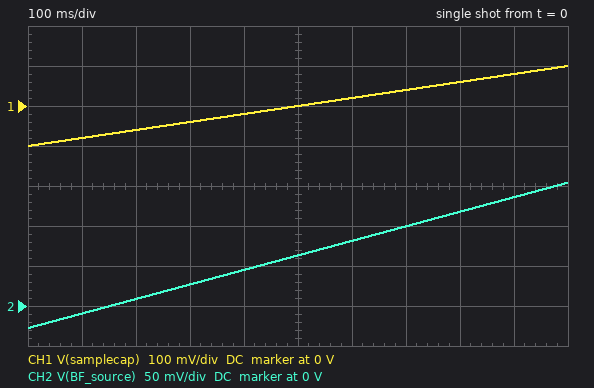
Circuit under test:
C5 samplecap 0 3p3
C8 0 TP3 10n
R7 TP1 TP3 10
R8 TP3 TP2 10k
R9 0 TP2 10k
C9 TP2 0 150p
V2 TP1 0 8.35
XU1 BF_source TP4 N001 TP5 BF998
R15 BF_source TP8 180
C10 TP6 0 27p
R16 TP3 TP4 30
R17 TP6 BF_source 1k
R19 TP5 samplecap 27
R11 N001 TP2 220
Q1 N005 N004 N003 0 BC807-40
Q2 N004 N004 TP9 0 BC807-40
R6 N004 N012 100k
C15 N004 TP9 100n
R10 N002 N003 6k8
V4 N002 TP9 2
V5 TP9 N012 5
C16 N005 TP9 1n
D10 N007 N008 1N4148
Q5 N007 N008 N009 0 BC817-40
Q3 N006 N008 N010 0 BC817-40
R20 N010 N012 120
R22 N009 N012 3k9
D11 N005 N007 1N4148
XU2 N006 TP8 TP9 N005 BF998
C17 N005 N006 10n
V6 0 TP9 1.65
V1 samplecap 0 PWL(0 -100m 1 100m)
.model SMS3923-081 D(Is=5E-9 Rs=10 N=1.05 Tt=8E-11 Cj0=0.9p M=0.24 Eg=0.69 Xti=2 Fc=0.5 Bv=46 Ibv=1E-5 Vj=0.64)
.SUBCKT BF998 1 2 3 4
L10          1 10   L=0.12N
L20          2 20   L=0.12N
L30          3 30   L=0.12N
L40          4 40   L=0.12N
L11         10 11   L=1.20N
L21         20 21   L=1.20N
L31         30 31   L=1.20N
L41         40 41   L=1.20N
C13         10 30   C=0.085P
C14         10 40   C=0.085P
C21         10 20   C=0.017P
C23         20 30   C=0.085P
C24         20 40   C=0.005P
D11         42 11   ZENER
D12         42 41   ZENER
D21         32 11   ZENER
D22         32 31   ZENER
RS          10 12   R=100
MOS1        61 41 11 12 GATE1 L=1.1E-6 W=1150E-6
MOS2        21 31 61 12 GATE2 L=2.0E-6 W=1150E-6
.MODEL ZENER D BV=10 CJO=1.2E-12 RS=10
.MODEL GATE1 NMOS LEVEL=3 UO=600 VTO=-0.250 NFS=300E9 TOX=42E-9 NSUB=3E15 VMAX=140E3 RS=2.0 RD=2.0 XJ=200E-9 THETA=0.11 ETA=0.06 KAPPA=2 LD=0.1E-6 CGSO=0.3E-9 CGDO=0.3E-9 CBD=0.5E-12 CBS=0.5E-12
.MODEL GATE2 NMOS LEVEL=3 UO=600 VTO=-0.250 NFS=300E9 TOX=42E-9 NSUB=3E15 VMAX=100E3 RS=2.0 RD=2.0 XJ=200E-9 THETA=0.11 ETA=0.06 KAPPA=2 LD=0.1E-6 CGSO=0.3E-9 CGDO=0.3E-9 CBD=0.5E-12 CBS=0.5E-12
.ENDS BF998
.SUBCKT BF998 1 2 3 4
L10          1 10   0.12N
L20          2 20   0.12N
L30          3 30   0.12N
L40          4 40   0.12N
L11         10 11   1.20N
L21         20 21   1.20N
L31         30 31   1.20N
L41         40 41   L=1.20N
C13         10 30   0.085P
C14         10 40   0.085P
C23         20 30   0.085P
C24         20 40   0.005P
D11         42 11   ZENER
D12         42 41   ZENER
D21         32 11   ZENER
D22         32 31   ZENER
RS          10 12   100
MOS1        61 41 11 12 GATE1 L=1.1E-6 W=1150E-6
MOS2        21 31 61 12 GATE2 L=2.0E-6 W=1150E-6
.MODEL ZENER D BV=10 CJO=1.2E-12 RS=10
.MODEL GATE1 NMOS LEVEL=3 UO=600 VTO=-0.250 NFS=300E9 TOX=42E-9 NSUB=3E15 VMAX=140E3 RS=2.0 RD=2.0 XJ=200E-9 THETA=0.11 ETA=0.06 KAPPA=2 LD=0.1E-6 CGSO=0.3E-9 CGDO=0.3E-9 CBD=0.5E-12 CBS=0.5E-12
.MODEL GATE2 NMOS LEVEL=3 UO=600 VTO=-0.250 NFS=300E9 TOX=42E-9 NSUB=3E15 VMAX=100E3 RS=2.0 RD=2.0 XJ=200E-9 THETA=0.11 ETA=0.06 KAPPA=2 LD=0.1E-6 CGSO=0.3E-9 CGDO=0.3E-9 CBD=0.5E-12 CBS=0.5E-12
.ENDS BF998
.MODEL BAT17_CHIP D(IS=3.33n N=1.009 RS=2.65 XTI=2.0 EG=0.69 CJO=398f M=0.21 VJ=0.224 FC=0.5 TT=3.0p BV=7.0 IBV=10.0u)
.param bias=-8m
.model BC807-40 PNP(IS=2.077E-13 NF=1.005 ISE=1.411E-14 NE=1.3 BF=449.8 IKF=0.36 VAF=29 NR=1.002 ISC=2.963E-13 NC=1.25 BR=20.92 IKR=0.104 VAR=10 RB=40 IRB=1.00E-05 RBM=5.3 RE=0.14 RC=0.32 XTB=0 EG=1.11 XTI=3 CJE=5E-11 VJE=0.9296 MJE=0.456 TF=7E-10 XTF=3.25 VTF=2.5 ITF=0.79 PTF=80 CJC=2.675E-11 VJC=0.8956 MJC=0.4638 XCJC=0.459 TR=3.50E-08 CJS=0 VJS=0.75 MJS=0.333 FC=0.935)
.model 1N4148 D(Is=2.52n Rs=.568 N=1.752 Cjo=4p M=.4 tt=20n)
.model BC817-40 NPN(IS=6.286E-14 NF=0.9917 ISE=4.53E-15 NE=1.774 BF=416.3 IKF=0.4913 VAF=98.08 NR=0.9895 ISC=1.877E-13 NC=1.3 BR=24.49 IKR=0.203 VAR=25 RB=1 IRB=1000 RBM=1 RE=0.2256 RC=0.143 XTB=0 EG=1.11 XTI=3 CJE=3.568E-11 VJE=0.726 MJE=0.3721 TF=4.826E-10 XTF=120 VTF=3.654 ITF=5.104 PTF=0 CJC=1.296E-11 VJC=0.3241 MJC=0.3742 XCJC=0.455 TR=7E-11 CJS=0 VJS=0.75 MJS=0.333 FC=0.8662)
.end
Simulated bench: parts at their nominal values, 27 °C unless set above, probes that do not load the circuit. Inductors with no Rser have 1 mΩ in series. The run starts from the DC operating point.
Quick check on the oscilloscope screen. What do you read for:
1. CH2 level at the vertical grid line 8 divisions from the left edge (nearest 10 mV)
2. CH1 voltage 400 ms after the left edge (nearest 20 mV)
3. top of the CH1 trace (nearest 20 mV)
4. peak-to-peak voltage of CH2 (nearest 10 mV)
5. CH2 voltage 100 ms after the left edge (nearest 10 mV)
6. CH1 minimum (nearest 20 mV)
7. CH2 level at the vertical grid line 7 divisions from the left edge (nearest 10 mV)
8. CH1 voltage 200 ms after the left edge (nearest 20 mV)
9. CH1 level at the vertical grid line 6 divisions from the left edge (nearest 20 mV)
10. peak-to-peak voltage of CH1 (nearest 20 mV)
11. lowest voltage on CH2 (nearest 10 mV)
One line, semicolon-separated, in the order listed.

120 mV; -20 mV; 100 mV; 180 mV; -10 mV; -100 mV; 100 mV; -60 mV; 20 mV; 200 mV; -30 mV
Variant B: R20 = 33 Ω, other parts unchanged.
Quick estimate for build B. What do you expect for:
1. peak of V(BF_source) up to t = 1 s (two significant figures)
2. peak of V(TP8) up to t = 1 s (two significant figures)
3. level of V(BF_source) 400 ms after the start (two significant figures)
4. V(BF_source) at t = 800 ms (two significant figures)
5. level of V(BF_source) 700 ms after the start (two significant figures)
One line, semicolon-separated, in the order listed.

-330 mV; -4.5 V; -440 mV; -370 mV; -390 mV
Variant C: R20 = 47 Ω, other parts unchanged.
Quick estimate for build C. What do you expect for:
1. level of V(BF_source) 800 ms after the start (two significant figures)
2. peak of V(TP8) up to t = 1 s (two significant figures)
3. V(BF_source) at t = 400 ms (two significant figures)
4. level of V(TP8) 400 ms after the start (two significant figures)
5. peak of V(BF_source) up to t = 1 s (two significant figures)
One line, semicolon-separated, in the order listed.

-210 mV; -3.3 V; -280 mV; -3.4 V; -170 mV
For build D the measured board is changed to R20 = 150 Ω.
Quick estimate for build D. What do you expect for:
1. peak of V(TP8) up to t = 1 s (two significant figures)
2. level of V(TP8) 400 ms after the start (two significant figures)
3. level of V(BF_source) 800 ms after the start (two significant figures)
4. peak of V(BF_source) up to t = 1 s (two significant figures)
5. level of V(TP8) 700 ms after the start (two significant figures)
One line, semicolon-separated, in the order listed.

-950 mV; -1.1 V; 180 mV; 210 mV; -1.0 V
